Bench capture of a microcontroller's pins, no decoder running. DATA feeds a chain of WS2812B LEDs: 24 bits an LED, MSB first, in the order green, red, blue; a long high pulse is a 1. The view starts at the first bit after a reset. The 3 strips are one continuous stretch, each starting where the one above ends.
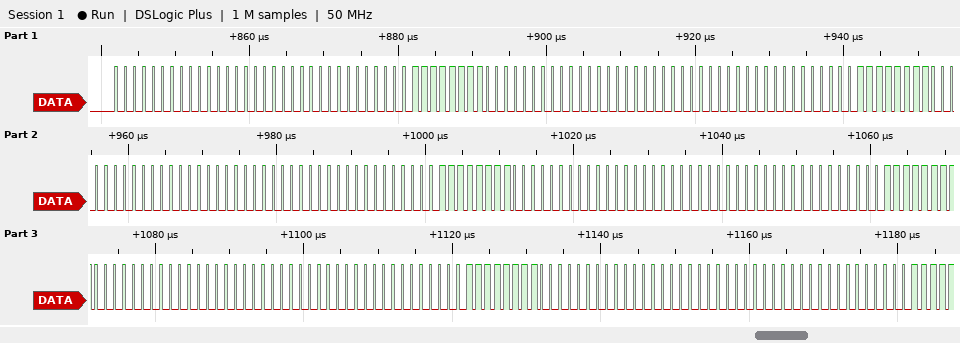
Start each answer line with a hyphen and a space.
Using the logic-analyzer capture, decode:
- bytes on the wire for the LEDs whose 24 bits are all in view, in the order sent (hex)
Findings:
- 00 00 00 00 FF 00 00 00 00 00 FF 00 00 00 00 00 FF 00 00 00 00 00 FF 00 00 00 00 00 FF 00 00 00 00
